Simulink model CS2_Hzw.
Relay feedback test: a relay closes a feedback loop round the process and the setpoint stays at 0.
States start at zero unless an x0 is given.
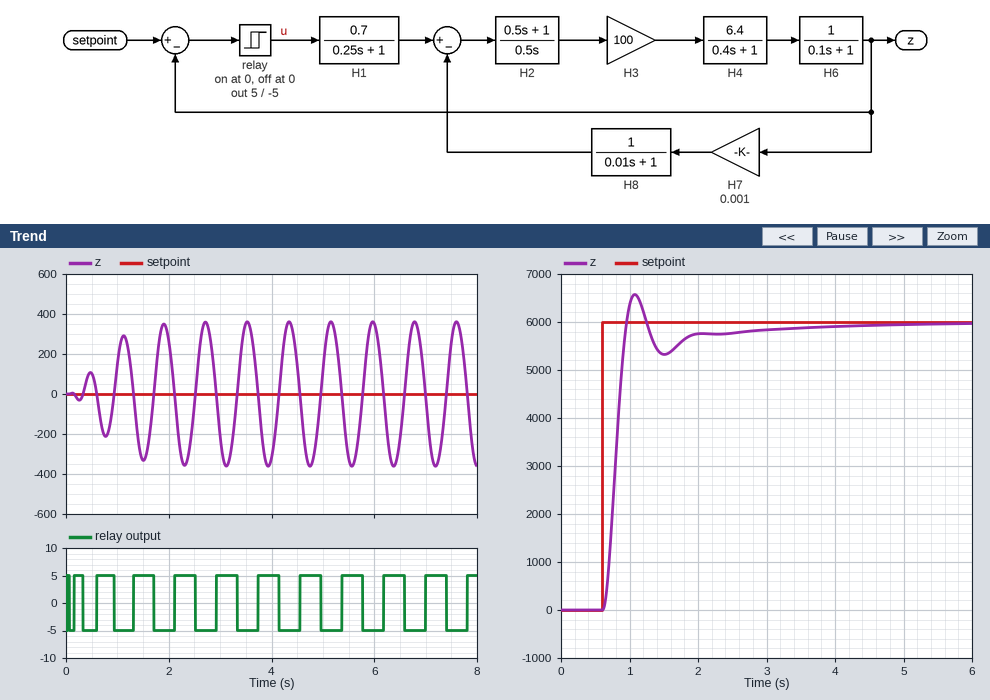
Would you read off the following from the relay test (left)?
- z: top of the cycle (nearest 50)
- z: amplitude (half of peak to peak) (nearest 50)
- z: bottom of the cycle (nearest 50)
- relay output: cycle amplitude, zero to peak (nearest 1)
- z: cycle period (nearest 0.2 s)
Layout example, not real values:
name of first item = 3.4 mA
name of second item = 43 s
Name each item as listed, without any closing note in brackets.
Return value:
z: top of the cycle = 350
z: amplitude (half of peak to peak) = 350
z: bottom of the cycle = -350
relay output: cycle amplitude, zero to peak = 5
z: cycle period = 0.8 s
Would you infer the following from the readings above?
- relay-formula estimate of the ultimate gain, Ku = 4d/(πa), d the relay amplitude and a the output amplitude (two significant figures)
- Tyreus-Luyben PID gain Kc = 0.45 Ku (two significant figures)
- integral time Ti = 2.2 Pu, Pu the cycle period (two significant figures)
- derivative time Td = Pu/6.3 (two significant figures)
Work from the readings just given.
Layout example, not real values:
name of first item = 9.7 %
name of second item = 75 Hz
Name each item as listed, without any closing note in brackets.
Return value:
relay-formula estimate of the ultimate gain, Ku = 4d/(πa), d the relay amplitude and a the output amplitude = 0.018
Tyreus-Luyben PID gain Kc = 0.45 Ku = 0.0081
integral time Ti = 2.2 Pu, Pu the cycle period = 1.8 s
derivative time Td = Pu/6.3 = 0.13 s
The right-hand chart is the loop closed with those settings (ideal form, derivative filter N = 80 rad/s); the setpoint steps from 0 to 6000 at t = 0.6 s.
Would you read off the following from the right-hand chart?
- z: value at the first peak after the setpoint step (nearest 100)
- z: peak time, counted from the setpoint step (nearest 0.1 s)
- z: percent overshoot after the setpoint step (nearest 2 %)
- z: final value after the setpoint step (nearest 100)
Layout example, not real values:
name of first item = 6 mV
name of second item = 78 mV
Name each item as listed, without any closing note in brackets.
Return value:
z: value at the first peak after the setpoint step = 6600
z: peak time, counted from the setpoint step = 0.5 s
z: percent overshoot after the setpoint step = 10 %
z: final value after the setpoint step = 6000
